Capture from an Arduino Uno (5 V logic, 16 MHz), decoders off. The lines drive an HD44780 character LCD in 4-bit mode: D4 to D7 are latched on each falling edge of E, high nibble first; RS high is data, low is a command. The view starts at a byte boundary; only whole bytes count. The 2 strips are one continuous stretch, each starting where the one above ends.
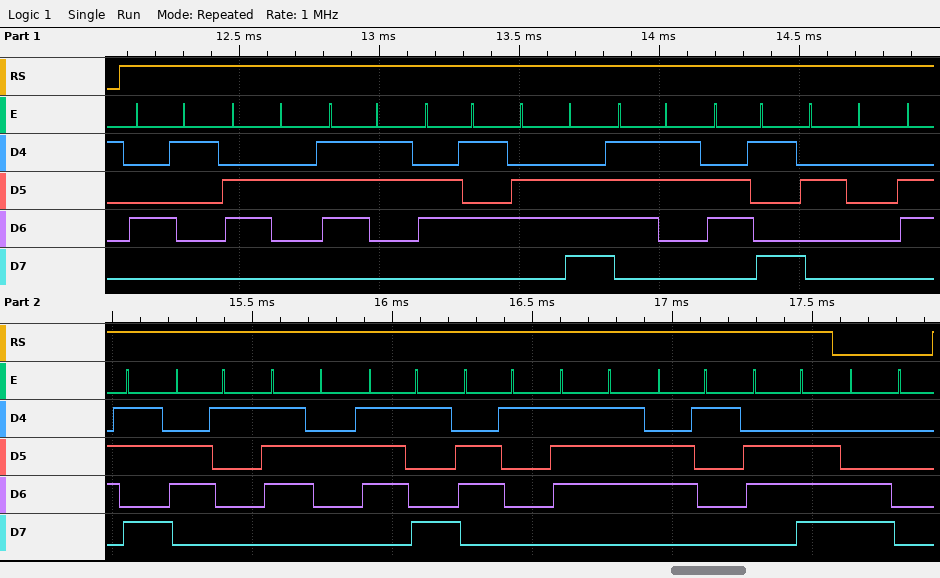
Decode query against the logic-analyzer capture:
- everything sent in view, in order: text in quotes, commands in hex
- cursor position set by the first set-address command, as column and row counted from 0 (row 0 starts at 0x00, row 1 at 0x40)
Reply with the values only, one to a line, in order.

"Absensi karyawan" 0xC0
column 0, row 1
